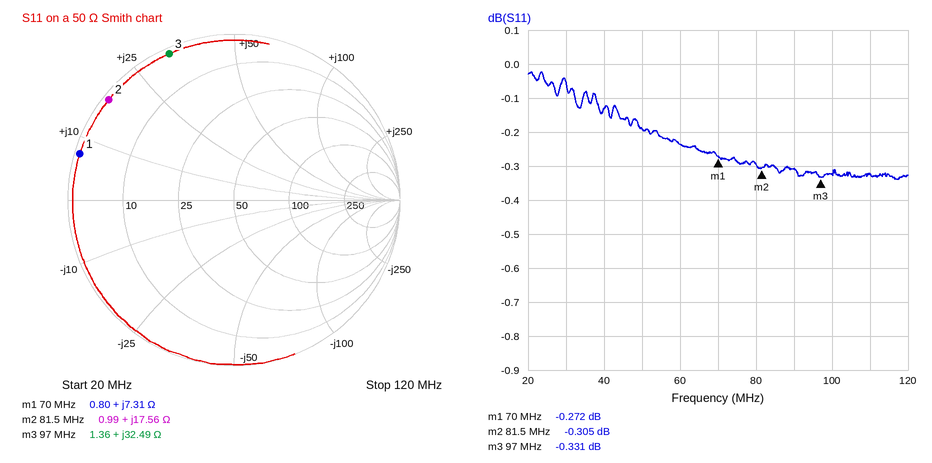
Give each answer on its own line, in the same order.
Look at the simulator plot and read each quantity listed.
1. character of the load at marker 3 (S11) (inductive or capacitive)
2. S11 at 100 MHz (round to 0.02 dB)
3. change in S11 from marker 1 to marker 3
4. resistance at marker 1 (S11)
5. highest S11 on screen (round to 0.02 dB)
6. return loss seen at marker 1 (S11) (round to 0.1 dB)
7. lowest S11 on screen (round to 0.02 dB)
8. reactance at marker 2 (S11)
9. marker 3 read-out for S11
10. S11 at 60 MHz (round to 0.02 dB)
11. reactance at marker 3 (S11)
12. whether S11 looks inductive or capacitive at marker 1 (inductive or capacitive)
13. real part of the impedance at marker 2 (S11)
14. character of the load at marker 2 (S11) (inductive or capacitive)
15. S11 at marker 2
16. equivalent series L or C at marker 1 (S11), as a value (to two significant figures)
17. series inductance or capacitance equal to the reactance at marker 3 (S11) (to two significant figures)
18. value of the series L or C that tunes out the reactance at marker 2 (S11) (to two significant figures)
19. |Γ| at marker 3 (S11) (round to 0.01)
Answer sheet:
inductive
-0.32 dB
-0.059 dB
0.80 Ω
-0.02 dB
0.3 dB
-0.34 dB
+17.56 Ω
-0.331 dB
-0.24 dB
+32.49 Ω
inductive
0.99 Ω
inductive
-0.305 dB
17 nH
53 nH
110 pF
0.96
